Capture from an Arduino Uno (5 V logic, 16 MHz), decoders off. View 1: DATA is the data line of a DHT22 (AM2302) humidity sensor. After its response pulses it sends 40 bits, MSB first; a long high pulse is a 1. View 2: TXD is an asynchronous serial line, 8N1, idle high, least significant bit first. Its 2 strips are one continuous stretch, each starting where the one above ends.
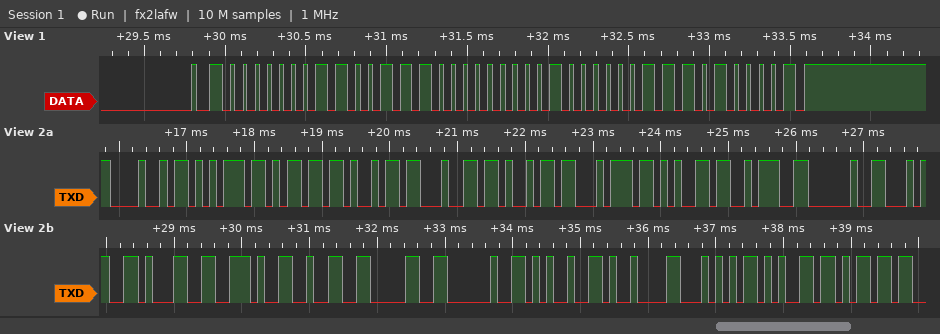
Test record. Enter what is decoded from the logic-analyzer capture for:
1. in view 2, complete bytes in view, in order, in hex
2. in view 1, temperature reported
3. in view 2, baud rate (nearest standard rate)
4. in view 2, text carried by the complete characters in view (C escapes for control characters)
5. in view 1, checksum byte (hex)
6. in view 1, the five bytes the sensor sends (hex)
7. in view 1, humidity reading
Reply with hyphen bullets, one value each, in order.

- 48 75 6D 69 64 69 74 65 3A 20 34 31 2E 32 30 20 25 09 54 65 6D
- 25.9 °C
- 9600 baud
- "Humidite: 41.20 %\tTem"
- 0xA1
- 01 9C 01 03 A1
- 41.2 %
